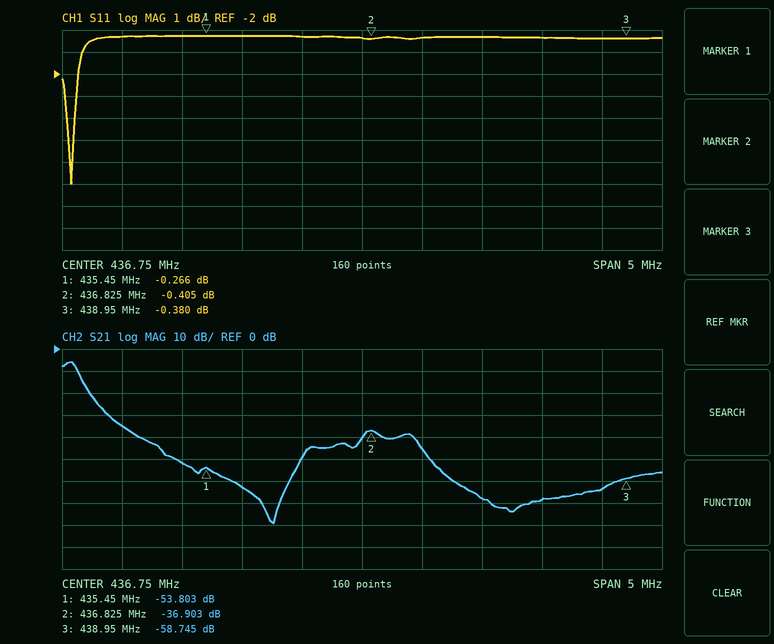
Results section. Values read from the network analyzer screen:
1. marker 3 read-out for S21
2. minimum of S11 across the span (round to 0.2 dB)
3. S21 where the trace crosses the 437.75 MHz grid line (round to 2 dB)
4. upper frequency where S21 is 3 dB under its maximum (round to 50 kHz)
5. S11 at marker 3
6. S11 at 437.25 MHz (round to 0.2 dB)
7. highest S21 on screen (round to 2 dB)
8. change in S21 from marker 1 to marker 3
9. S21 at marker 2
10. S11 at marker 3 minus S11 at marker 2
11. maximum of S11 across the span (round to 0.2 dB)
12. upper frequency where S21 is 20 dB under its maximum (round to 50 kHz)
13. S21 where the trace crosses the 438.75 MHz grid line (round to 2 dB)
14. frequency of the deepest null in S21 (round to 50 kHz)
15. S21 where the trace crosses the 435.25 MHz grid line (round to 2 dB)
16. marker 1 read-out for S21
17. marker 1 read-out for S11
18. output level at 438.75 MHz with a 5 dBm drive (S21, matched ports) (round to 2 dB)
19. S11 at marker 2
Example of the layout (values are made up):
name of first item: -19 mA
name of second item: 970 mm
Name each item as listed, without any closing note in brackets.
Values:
marker 3 read-out for S21: -58.745 dB
minimum of S11 across the span: -7.0 dB
S21 where the trace crosses the 437.75 MHz grid line: -68 dB
upper frequency where S21 is 3 dB under its maximum: 434.35 MHz
S11 at marker 3: -0.380 dB
S11 at 437.25 MHz: -0.4 dB
highest S21 on screen: -6 dB
change in S21 from marker 1 to marker 3: -4.942 dB
S21 at marker 2: -36.903 dB
S11 at marker 3 minus S11 at marker 2: 0.025 dB
maximum of S11 across the span: -0.2 dB
upper frequency where S21 is 20 dB under its maximum: 434.55 MHz
S21 where the trace crosses the 438.75 MHz grid line: -64 dB
frequency of the deepest null in S21: 436.00 MHz
S21 where the trace crosses the 435.25 MHz grid line: -52 dB
marker 1 read-out for S21: -53.803 dB
marker 1 read-out for S11: -0.266 dB
output level at 438.75 MHz with a 5 dBm drive (S21, matched ports): -58 dBm
S11 at marker 2: -0.405 dB
